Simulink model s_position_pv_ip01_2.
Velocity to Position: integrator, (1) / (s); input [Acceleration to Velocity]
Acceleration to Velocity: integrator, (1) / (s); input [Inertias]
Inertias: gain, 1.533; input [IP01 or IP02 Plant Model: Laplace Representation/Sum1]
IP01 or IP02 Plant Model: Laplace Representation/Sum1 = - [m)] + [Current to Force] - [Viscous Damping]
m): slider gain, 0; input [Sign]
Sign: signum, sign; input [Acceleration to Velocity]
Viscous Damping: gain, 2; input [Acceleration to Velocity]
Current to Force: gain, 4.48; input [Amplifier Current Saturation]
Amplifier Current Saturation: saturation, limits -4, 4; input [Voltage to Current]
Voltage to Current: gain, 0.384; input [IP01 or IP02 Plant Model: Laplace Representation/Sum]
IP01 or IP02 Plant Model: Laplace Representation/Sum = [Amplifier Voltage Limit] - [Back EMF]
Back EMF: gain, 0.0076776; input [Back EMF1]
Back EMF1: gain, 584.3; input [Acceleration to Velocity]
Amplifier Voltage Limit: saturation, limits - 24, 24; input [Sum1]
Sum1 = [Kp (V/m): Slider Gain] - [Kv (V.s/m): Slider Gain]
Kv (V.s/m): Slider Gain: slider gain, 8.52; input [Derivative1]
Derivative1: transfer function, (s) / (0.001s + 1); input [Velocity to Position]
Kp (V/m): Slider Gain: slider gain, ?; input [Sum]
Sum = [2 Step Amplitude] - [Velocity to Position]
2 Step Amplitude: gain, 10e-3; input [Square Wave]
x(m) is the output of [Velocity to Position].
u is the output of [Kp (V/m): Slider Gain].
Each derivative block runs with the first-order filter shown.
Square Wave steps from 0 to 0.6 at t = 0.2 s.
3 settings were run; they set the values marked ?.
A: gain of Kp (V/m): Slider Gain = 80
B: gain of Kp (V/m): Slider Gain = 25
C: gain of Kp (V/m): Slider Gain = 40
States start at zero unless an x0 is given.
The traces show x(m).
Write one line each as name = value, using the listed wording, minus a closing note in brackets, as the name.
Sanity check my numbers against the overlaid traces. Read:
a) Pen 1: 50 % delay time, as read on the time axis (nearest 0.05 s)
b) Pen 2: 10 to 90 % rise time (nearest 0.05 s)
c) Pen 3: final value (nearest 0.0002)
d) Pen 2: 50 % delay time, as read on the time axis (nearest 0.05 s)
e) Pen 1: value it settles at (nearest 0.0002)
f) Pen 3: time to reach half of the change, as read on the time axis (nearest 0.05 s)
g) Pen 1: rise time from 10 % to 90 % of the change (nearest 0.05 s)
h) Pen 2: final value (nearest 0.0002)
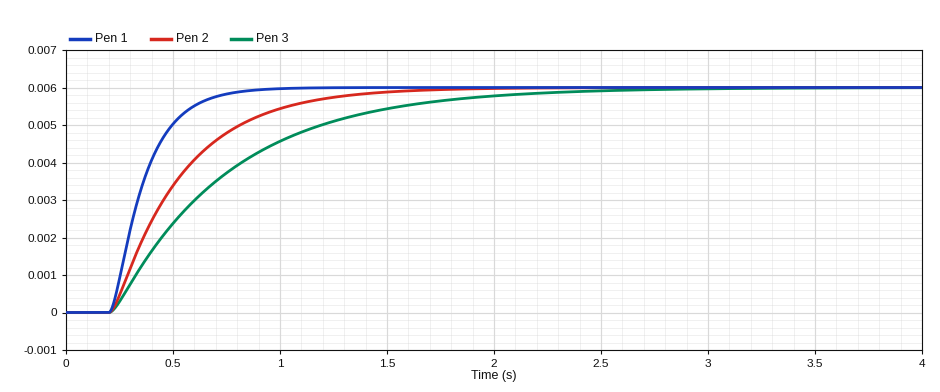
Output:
Pen 1: 50 % delay time, as read on the time axis = 0.35 s
Pen 2: 10 to 90 % rise time = 0.70 s
Pen 3: final value = 0.0060
Pen 2: 50 % delay time, as read on the time axis = 0.45 s
Pen 1: value it settles at = 0.0060
Pen 3: time to reach half of the change, as read on the time axis = 0.60 s
Pen 1: rise time from 10 % to 90 % of the change = 0.35 s
Pen 2: final value = 0.0060
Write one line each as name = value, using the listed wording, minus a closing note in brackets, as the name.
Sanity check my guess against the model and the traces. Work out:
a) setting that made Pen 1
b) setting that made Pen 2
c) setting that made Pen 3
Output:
setting that made Pen 1 = A
setting that made Pen 2 = C
setting that made Pen 3 = B
